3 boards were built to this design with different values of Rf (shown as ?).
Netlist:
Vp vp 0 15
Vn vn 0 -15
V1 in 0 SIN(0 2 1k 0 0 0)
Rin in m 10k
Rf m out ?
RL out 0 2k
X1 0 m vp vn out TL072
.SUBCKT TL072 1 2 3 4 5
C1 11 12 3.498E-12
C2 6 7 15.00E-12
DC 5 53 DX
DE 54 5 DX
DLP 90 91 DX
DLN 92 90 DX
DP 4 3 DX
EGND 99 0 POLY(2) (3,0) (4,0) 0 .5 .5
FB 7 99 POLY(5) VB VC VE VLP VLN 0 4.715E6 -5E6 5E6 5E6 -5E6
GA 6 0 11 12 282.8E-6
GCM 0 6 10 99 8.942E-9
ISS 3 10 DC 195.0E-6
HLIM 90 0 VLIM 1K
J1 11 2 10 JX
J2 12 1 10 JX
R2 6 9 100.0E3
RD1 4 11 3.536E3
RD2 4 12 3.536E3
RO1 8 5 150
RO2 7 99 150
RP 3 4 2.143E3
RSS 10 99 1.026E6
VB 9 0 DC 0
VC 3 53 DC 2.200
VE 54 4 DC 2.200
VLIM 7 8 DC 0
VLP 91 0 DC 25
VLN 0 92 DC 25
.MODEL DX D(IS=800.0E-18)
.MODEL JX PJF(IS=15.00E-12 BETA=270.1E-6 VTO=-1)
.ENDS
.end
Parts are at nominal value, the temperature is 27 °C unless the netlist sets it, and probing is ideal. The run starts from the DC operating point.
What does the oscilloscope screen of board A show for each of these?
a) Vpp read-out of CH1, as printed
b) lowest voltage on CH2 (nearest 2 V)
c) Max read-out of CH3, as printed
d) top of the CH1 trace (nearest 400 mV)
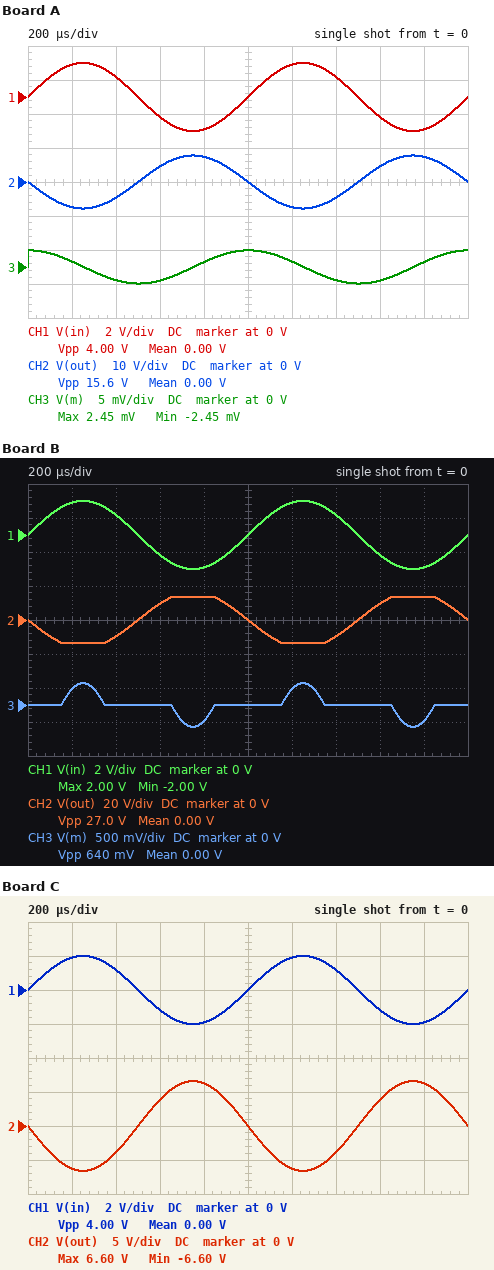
4.00 V
-8 V
2.45 mV
2.0 V
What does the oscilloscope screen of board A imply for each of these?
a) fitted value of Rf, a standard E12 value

39 kΩ
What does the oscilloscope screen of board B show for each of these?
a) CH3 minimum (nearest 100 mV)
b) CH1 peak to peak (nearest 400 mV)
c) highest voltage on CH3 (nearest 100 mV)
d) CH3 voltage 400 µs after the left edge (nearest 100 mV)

-300 mV
4.0 V
300 mV
0 V
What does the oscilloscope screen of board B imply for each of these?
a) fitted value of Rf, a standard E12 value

82 kΩ
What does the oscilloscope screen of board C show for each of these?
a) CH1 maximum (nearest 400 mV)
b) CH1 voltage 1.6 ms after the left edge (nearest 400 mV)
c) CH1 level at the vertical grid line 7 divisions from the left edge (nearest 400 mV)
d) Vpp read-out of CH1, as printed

2.0 V
-1.2 V
1.2 V
4.00 V
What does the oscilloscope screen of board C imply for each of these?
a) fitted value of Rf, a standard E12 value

33 kΩ
